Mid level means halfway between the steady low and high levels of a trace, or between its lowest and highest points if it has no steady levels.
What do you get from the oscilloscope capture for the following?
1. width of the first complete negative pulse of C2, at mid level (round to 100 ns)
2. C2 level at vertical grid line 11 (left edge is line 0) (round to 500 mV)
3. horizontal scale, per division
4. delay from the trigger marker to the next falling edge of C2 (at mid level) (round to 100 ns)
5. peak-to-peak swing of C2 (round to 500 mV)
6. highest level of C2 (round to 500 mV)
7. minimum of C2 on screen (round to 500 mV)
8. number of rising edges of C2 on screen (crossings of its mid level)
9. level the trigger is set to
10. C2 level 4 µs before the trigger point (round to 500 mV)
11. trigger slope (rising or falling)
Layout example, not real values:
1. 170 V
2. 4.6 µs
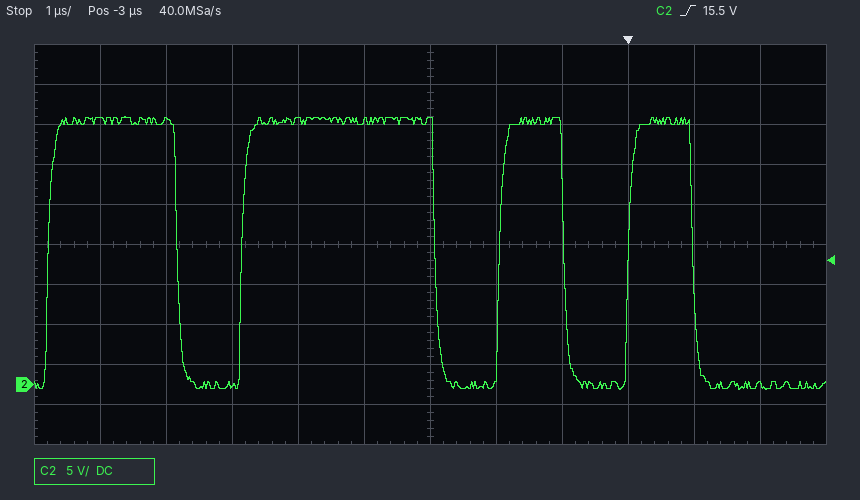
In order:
1. 1.0 µs
2. 0.0 V
3. 1 µs
4. 1.0 µs
5. 34.0 V
6. 33.5 V
7. -500 mV
8. 4
9. 15.5 V
10. 33.0 V
11. rising
